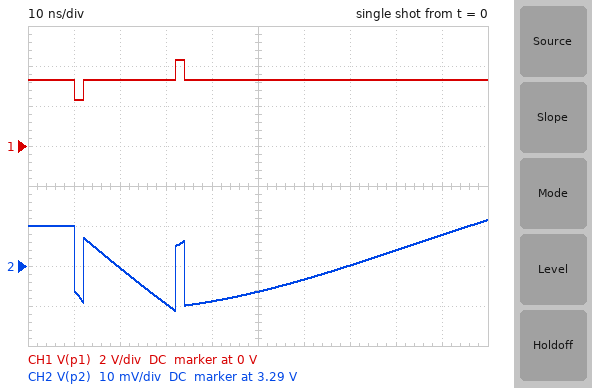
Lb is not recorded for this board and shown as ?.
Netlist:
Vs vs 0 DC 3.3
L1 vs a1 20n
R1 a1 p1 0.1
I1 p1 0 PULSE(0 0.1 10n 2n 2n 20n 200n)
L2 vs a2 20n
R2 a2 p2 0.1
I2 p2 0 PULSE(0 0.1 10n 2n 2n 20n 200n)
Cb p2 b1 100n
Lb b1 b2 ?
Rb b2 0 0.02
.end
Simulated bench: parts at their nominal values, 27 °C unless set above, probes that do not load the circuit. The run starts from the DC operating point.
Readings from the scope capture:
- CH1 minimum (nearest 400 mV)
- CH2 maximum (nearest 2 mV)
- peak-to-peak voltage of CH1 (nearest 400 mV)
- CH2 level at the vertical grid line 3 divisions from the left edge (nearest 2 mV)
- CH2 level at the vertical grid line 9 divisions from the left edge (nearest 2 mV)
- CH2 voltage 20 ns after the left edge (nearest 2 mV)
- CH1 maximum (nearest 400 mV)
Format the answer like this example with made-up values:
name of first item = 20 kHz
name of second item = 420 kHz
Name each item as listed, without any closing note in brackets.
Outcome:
CH1 minimum = 2.4 V
CH2 maximum = 3.302 V
peak-to-peak voltage of CH1 = 2.0 V
CH2 level at the vertical grid line 3 divisions from the left edge = 3.280 V
CH2 level at the vertical grid line 9 divisions from the left edge = 3.298 V
CH2 voltage 20 ns after the left edge = 3.290 V
CH1 maximum = 4.4 V
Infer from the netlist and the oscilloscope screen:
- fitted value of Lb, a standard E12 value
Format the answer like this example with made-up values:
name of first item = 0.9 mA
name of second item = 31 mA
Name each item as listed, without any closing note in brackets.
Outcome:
fitted value of Lb, a standard E12 value = 330 pH
